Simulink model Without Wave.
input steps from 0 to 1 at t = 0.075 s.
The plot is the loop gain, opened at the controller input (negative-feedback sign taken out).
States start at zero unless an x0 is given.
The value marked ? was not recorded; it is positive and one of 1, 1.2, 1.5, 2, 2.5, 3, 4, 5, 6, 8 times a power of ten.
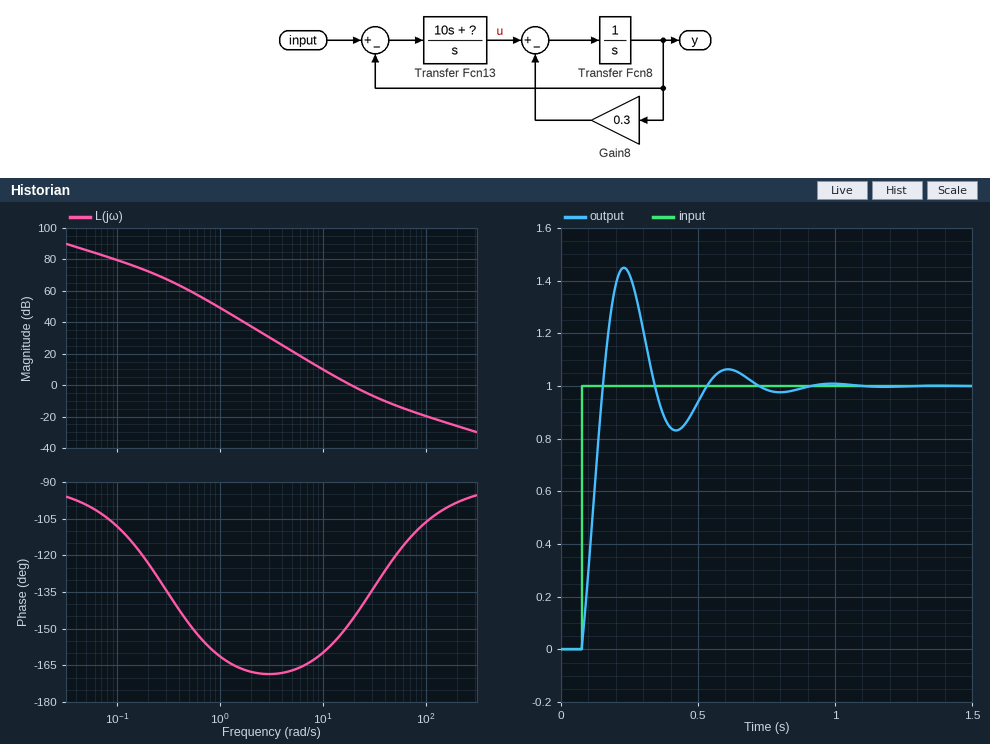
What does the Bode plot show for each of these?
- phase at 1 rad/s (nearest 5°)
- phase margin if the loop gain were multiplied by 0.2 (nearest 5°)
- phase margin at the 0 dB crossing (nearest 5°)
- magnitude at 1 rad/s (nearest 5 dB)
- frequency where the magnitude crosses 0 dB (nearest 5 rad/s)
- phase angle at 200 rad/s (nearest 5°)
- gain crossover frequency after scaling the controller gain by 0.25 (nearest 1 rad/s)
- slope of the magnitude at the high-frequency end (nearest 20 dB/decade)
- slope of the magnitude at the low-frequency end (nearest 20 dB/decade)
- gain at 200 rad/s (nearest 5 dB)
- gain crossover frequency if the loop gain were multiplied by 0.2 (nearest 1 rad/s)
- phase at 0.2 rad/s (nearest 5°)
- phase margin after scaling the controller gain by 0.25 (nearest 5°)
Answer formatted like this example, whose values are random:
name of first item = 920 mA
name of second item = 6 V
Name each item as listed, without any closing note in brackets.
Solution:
phase at 1 rad/s = -160°
phase margin if the loop gain were multiplied by 0.2 = 15°
phase margin at the 0 dB crossing = 35°
magnitude at 1 rad/s = 50 dB
frequency where the magnitude crosses 0 dB = 20 rad/s
phase angle at 200 rad/s = -100°
gain crossover frequency after scaling the controller gain by 0.25 = 9 rad/s
slope of the magnitude at the high-frequency end = -20 dB/decade
slope of the magnitude at the low-frequency end = -20 dB/decade
gain at 200 rad/s = -25 dB
gain crossover frequency if the loop gain were multiplied by 0.2 = 8 rad/s
phase at 0.2 rad/s = -125°
phase margin after scaling the controller gain by 0.25 = 20°
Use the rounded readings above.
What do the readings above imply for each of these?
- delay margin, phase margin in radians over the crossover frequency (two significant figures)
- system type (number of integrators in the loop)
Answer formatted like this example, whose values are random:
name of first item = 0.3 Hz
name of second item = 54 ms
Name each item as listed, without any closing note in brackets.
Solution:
delay margin, phase margin in radians over the crossover frequency = 0.031 s
system type = 1
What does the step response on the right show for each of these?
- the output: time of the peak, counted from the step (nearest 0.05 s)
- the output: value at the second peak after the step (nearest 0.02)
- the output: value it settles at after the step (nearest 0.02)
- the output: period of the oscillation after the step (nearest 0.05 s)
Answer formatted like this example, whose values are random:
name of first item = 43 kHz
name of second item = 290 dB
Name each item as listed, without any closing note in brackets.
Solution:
the output: time of the peak, counted from the step = 0.15 s
the output: value at the second peak after the step = 1.06
the output: value it settles at after the step = 1.00
the output: period of the oscillation after the step = 0.40 s
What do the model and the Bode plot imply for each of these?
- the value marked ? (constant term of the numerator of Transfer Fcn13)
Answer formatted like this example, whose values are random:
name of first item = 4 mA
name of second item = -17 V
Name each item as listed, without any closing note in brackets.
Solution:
the value marked ? = 300
